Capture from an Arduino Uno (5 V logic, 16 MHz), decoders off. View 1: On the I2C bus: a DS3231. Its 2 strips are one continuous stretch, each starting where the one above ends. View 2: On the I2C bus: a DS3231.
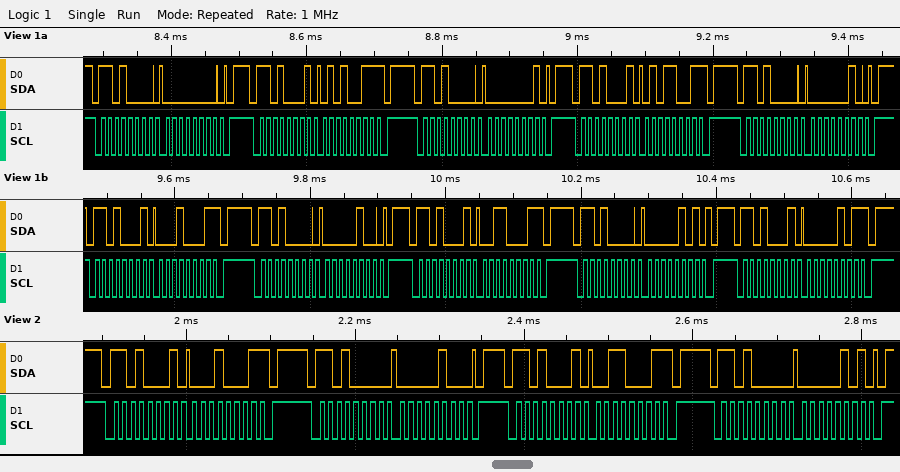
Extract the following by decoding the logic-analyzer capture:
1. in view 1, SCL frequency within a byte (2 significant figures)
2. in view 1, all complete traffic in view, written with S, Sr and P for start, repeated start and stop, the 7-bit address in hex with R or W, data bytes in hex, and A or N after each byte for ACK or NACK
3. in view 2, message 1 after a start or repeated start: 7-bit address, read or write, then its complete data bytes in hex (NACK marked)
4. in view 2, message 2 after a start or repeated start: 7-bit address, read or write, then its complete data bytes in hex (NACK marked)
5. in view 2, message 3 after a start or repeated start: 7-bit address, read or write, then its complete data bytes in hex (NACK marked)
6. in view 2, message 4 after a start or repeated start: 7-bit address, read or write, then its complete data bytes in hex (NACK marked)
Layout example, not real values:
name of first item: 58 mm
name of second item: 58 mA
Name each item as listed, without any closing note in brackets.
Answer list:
in view 1, SCL frequency within a byte: 100 kHz
in view 1, all complete traffic in view, written with S, Sr and P for start, repeated start and stop, the 7-bit address in hex with R or W, data bytes in hex, and A or N after each byte for ACK or NACK: S 68W A 00 A P S 68R A 53 N P S 68W A 01 A P S 68R A 59 N P S 68W A 02 A P S 68R A 11 N P S 68W A 04 A P S 68R A 31 N P S 68W A 05 A P S 68R A 05 N P
in view 2, message 1 after a start or repeated start: 7-bit address, read or write, then its complete data bytes in hex: 0x68 read: 11 NACK
in view 2, message 2 after a start or repeated start: 7-bit address, read or write, then its complete data bytes in hex: 0x68 write: 04
in view 2, message 3 after a start or repeated start: 7-bit address, read or write, then its complete data bytes in hex: 0x68 read: 31 NACK
in view 2, message 4 after a start or repeated start: 7-bit address, read or write, then its complete data bytes in hex: 0x68 write: 05
